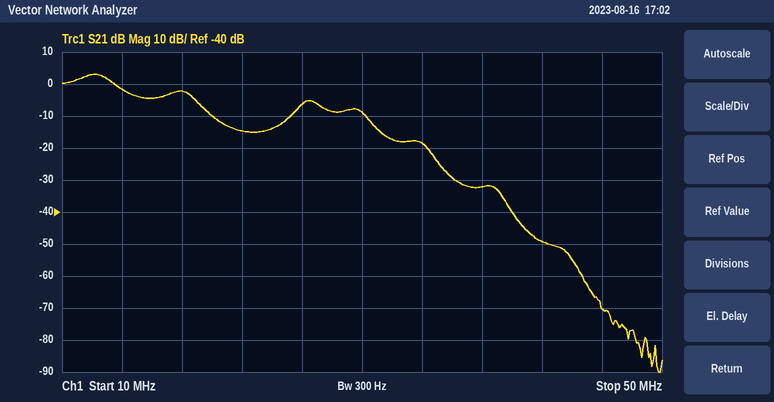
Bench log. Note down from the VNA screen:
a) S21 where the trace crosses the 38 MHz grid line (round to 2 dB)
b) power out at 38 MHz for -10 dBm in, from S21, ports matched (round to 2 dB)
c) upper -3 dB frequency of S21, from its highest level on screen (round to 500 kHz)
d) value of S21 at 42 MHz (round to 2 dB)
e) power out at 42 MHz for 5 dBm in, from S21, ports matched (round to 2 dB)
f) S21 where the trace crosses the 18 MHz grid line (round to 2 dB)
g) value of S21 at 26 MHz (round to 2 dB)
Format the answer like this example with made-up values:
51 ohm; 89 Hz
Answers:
-32 dB; -42 dBm; 13.5 MHz; -50 dB; -44 dBm; -2 dB; -6 dB
